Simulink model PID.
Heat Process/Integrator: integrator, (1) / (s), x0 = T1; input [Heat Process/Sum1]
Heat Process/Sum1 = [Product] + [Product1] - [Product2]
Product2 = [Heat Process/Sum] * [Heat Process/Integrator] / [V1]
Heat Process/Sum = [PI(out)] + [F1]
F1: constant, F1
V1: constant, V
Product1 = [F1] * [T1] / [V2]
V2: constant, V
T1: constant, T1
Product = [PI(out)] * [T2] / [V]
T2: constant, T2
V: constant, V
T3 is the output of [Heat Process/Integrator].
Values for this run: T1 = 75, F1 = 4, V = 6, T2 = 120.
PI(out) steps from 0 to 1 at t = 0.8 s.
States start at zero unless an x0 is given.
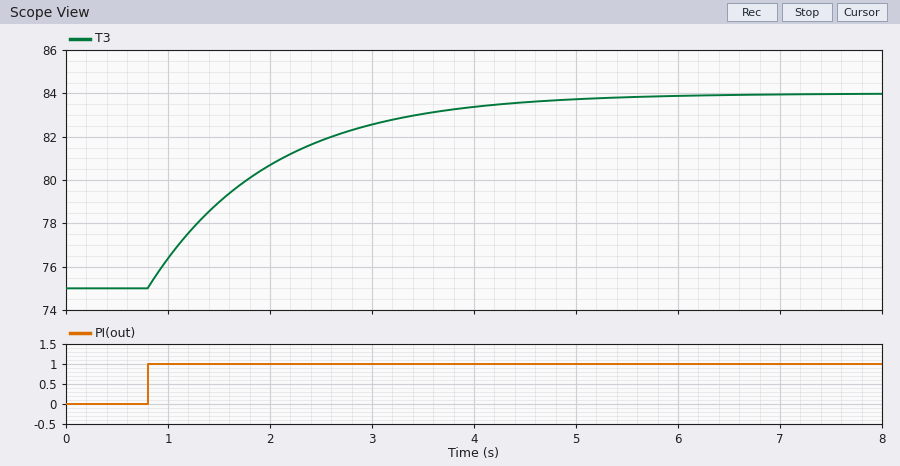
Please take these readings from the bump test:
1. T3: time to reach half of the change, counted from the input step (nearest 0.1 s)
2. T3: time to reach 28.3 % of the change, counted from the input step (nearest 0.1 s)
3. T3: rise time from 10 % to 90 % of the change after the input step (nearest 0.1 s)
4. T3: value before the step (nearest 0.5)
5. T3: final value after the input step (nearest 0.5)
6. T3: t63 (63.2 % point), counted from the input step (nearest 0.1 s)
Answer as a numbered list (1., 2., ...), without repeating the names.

1. 0.8 s
2. 0.4 s
3. 2.6 s
4. 75.0
5. 84.0
6. 1.2 s
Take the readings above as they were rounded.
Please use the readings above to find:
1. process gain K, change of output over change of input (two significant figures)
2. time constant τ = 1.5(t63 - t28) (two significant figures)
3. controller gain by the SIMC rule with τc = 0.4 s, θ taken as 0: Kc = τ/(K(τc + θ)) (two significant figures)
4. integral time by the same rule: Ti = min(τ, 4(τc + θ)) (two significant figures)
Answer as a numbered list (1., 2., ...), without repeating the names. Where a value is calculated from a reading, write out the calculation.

1. (84 - 75) / 1 = 9.0
2. 1.5 × (1.2 - 0.4) = 1.2 s
3. 1.2 / (9 × (0.4 + 0)) = 0.33
4. min(1.2, 4 × (0.4 + 0)) = 1.2 s
